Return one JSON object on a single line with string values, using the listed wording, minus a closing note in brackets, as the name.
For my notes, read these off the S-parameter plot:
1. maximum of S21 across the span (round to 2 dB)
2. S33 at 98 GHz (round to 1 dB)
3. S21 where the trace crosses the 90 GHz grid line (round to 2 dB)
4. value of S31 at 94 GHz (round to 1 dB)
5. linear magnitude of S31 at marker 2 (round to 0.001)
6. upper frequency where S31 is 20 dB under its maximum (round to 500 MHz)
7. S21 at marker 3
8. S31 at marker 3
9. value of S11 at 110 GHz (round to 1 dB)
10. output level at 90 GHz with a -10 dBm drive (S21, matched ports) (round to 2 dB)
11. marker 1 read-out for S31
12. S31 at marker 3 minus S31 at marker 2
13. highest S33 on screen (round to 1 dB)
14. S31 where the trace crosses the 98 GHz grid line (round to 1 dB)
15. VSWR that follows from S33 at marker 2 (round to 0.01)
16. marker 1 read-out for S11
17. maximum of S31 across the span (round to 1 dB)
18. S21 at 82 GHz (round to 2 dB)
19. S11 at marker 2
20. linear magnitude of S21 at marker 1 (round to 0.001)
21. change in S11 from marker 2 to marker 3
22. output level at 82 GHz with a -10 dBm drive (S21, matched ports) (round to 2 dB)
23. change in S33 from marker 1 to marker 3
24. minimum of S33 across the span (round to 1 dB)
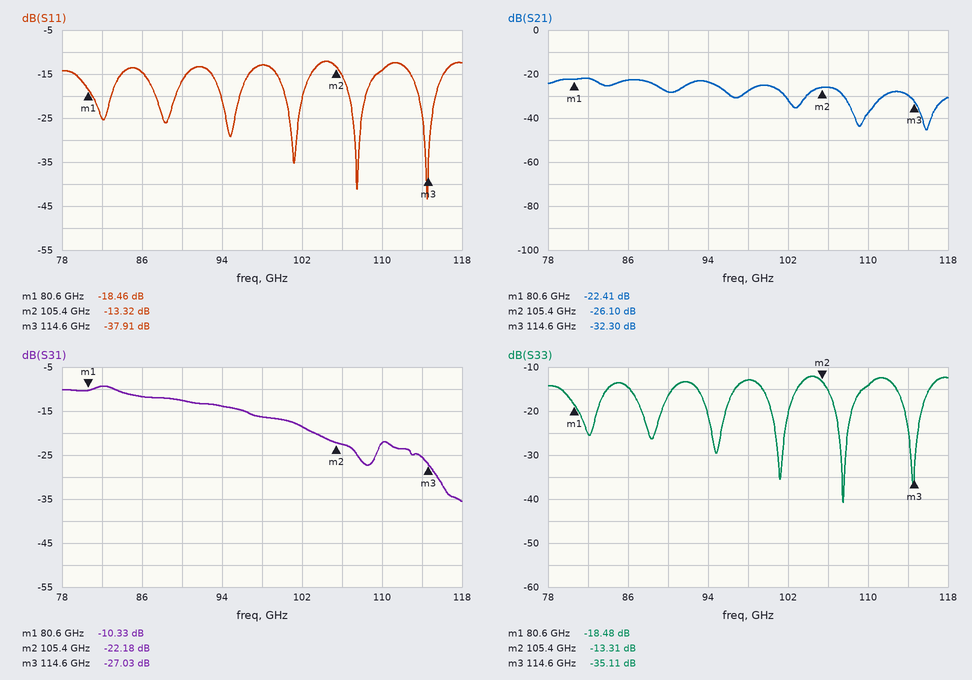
{"maximum of S21 across the span": "-22 dB", "S33 at 98 GHz": "-13 dB", "S21 where the trace crosses the 90 GHz grid line": "-28 dB", "value of S31 at 94 GHz": "-14 dB", "linear magnitude of S31 at marker 2": "0.078", "upper frequency where S31 is 20 dB under its maximum": "115.5 GHz", "S21 at marker 3": "-32.30 dB", "S31 at marker 3": "-27.03 dB", "value of S11 at 110 GHz": "-14 dB", "output level at 90 GHz with a -10 dBm drive (S21, matched ports)": "-38 dBm", "marker 1 read-out for S31": "-10.33 dB", "S31 at marker 3 minus S31 at marker 2": "-4.85 dB", "highest S33 on screen": "-12 dB", "S31 where the trace crosses the 98 GHz grid line": "-16 dB", "VSWR that follows from S33 at marker 2": "1.55", "marker 1 read-out for S11": "-18.46 dB", "maximum of S31 across the span": "-9 dB", "S21 at 82 GHz": "-22 dB", "S11 at marker 2": "-13.32 dB", "linear magnitude of S21 at marker 1": "0.076", "change in S11 from marker 2 to marker 3": "-24.59 dB", "output level at 82 GHz with a -10 dBm drive (S21, matched ports)": "-32 dBm", "change in S33 from marker 1 to marker 3": "-16.63 dB", "minimum of S33 across the span": "-41 dB"}
